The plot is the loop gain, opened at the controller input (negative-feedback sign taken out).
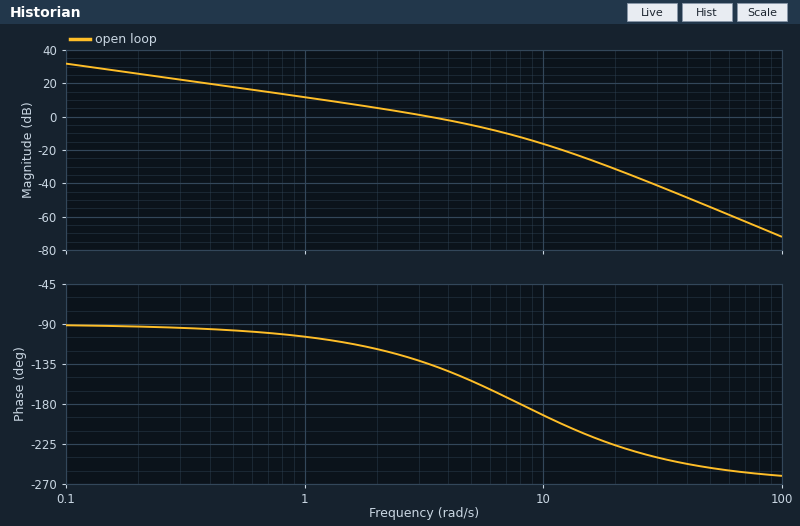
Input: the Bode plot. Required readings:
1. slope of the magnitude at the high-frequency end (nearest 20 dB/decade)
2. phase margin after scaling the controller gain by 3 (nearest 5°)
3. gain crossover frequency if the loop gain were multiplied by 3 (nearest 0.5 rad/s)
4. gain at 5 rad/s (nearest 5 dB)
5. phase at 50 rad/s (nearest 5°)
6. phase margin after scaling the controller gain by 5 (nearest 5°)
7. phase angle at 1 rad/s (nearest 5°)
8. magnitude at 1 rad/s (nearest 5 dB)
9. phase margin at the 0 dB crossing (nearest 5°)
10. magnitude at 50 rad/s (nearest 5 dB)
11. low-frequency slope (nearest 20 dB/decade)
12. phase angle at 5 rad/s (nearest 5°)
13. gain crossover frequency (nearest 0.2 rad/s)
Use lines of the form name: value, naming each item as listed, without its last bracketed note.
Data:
slope of the magnitude at the high-frequency end: -60 dB/decade
phase margin after scaling the controller gain by 3: 10°
gain crossover frequency if the loop gain were multiplied by 3: 7.0 rad/s
gain at 5 rad/s: -5 dB
phase at 50 rad/s: -250°
phase margin after scaling the controller gain by 5: -5°
phase angle at 1 rad/s: -105°
magnitude at 1 rad/s: 10 dB
phase margin at the 0 dB crossing: 45°
magnitude at 50 rad/s: -55 dB
low-frequency slope: -20 dB/decade
phase angle at 5 rad/s: -155°
gain crossover frequency: 3.4 rad/s
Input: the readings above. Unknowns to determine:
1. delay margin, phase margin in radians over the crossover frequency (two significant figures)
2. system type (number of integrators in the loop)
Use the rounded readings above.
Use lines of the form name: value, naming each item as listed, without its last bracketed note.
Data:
delay margin, phase margin in radians over the crossover frequency: 0.23 s
system type: 1
